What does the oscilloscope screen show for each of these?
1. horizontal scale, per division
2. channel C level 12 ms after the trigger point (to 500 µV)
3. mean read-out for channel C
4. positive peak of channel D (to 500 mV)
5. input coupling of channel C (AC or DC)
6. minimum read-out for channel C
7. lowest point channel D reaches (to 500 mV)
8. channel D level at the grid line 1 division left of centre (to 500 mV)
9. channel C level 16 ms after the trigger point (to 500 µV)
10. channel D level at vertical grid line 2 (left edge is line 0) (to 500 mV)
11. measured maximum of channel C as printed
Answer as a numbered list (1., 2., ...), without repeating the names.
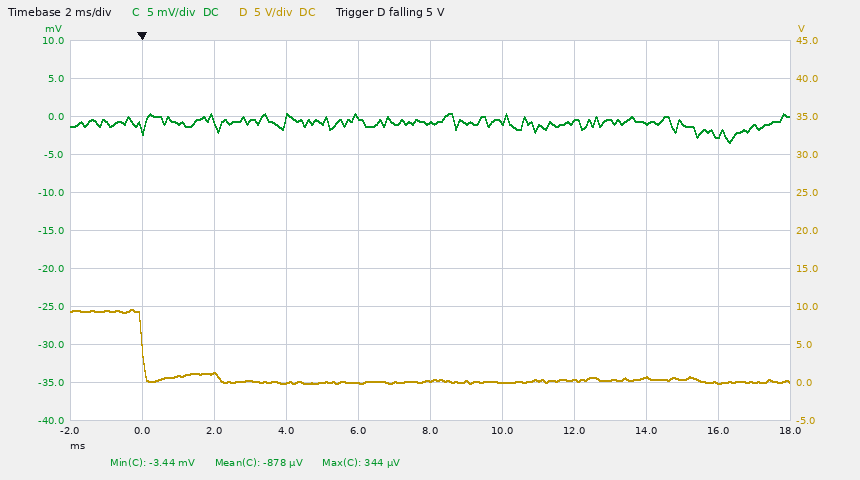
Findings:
1. 2 ms
2. -500 µV
3. -878 µV
4. 9.5 V
5. DC
6. -3.44 mV
7. 0.0 V
8. 0.0 V
9. -2.5 mV
10. 1.0 V
11. 344 µV
